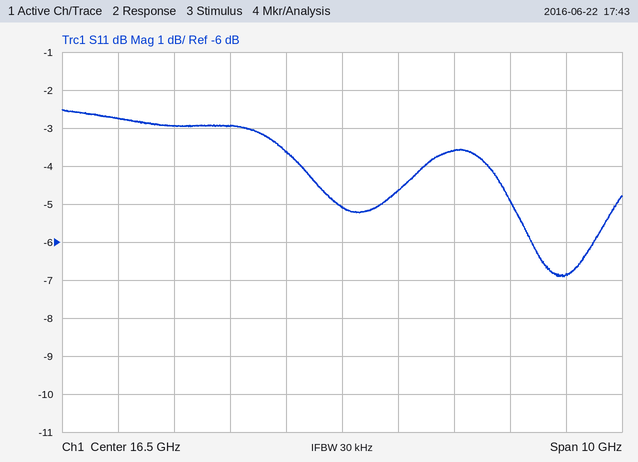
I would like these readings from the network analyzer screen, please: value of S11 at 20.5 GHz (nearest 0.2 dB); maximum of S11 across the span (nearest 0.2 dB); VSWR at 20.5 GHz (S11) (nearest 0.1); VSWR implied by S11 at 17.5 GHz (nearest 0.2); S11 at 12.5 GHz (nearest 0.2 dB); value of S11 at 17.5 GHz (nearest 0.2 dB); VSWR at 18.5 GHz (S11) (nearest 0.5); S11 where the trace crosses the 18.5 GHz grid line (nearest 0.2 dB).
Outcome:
-6.8 dB
-2.6 dB
2.7
3.8
-2.8 dB
-4.6 dB
5.0
-3.6 dB
